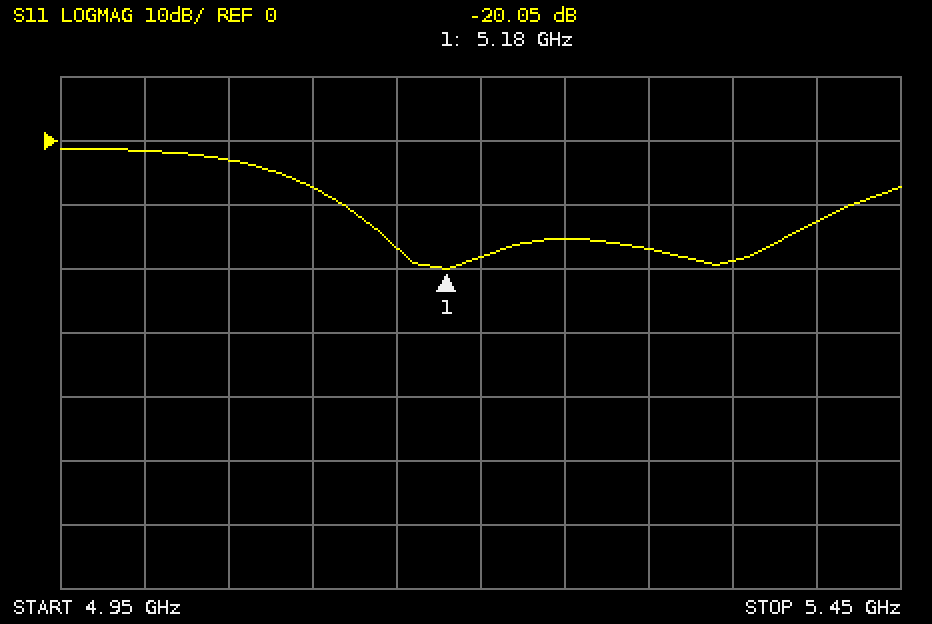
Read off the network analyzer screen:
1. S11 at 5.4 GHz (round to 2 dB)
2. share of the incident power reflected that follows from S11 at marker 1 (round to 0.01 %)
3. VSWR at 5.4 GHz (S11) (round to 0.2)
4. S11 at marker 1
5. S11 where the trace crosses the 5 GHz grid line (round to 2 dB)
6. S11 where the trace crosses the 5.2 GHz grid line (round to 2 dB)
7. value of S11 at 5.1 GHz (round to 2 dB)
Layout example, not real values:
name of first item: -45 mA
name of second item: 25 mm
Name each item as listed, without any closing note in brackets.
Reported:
S11 at 5.4 GHz: -12 dB
share of the incident power reflected that follows from S11 at marker 1: 0.99 %
VSWR at 5.4 GHz (S11): 1.6
S11 at marker 1: -20.05 dB
S11 where the trace crosses the 5 GHz grid line: -2 dB
S11 where the trace crosses the 5.2 GHz grid line: -18 dB
value of S11 at 5.1 GHz: -8 dB
